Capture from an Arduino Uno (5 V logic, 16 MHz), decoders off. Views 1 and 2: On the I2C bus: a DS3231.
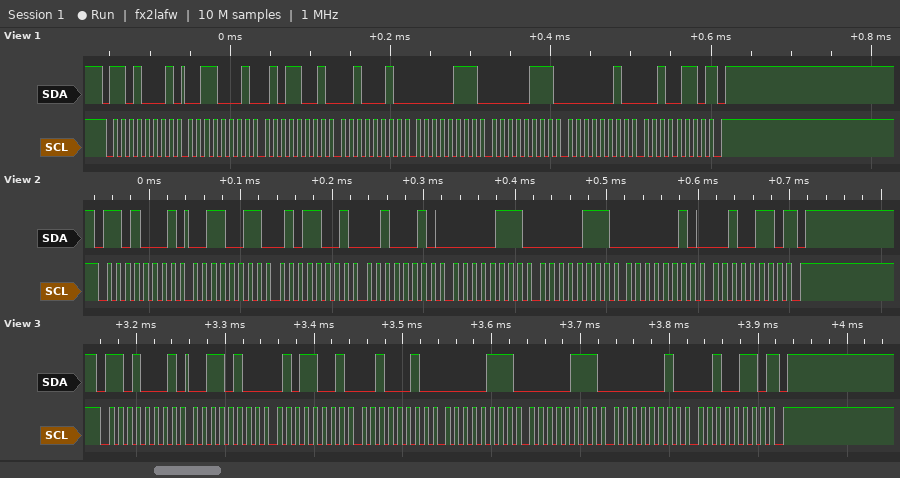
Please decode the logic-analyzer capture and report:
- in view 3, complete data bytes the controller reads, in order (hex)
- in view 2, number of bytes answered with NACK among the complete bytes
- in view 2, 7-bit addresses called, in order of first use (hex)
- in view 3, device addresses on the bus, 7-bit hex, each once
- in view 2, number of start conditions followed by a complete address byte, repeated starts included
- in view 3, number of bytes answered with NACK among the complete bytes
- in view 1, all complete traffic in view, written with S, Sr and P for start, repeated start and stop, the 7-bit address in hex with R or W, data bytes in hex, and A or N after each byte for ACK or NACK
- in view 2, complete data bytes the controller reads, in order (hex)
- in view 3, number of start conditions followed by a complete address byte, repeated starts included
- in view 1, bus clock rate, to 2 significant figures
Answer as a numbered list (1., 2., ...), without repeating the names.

1. 34 59 22 07 07 02 26
2. 1
3. 0x68
4. 0x68
5. 1
6. 1
7. S 68R A 31 A 59 A 22 A 07 A 07 A 02 A 26 N P
8. 33 59 22 07 07 02 26
9. 1
10. 100 kHz
